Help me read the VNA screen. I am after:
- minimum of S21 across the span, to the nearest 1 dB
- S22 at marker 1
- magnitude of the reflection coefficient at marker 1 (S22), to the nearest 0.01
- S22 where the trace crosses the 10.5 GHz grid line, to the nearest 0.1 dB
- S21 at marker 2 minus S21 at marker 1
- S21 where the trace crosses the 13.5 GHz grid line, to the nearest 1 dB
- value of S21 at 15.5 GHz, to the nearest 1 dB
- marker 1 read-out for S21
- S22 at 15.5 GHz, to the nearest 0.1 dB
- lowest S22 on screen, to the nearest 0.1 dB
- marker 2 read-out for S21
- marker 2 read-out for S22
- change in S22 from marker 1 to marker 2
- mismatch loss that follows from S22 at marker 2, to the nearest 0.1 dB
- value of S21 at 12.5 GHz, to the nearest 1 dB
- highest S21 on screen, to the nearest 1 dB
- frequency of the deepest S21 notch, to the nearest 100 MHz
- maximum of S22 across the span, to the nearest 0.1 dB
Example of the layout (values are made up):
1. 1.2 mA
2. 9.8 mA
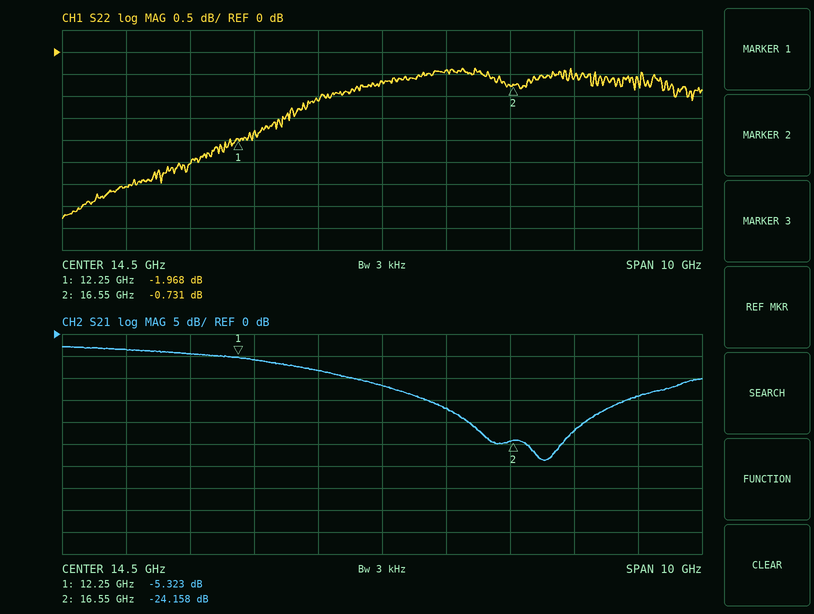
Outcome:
1. -29 dB
2. -1.968 dB
3. 0.80
4. -3.1 dB
5. -18.835 dB
6. -8 dB
7. -17 dB
8. -5.323 dB
9. -0.4 dB
10. -3.8 dB
11. -24.158 dB
12. -0.731 dB
13. 1.237 dB
14. 8.1 dB
15. -6 dB
16. -3 dB
17. 17.0 GHz
18. -0.4 dB
